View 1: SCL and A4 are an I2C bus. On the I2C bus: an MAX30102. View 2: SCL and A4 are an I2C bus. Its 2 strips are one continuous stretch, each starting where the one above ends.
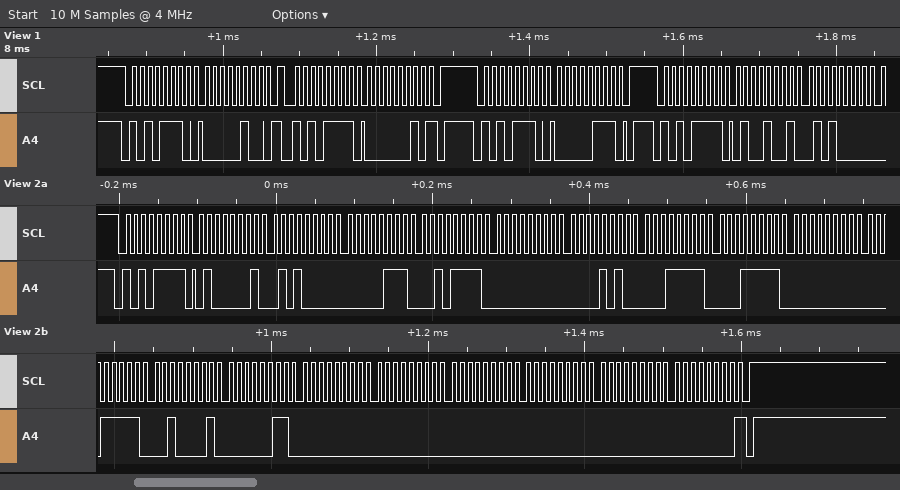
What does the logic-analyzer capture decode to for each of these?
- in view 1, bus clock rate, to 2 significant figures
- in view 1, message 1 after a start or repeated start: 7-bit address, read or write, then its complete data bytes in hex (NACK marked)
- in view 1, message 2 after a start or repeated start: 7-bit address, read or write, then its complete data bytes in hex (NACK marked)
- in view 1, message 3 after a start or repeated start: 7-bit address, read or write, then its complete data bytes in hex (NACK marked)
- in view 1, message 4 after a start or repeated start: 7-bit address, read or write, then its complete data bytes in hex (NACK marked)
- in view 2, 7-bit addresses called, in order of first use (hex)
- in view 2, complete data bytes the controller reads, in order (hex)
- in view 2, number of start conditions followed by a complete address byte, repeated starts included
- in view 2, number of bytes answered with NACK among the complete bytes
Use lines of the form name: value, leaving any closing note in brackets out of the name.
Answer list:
in view 1, bus clock rate, to 2 significant figures: 100 kHz
in view 1, message 1 after a start or repeated start: 7-bit address, read or write, then its complete data bytes in hex: 0x57 write: 04
in view 1, message 2 after a start or repeated start: 7-bit address, read or write, then its complete data bytes in hex: 0x57 read: 02 NACK
in view 1, message 3 after a start or repeated start: 7-bit address, read or write, then its complete data bytes in hex: 0x57 write: 07
in view 1, message 4 after a start or repeated start: 7-bit address, read or write, then its complete data bytes in hex: 0x57 read: 49 50
in view 2, 7-bit addresses called, in order of first use: 0x57
in view 2, complete data bytes the controller reads, in order: 41 50 07 2F 00 0A 1F 1F 00 1F 21 03 00 00 00 00 00 00
in view 2, number of start conditions followed by a complete address byte, repeated starts included: 1
in view 2, number of bytes answered with NACK among the complete bytes: 1
